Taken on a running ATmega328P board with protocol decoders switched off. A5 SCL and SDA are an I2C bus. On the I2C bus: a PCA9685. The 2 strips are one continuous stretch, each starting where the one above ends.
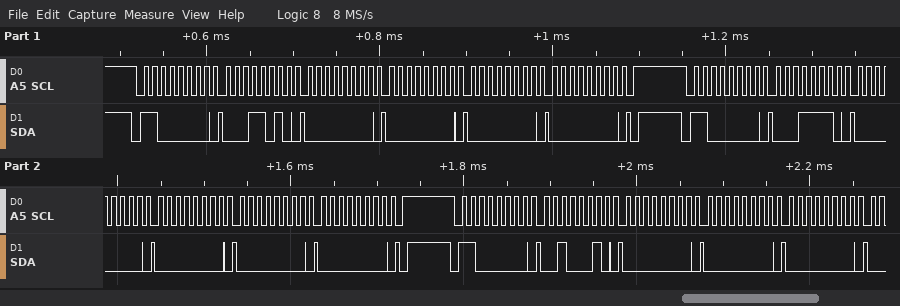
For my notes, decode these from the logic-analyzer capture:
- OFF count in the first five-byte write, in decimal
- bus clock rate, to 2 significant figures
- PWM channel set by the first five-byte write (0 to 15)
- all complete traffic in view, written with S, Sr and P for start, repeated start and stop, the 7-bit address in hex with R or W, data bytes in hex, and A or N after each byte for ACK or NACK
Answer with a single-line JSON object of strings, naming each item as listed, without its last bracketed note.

{"OFF count in the first five-byte write, in decimal": "0", "bus clock rate, to 2 significant figures": "100 kHz", "PWM channel set by the first five-byte write": "5", "all complete traffic in view, written with S, Sr and P for start, repeated start and stop, the 7-bit address in hex with R or W, data bytes in hex, and A or N after each byte for ACK or NACK": "S 60W A 1A A 00 A 00 A 00 A 00 A P S 60W A 1E A 00 A 00 A 00 A 00 A P S 60W A 22 A 00 A 00 A 00 A"}
